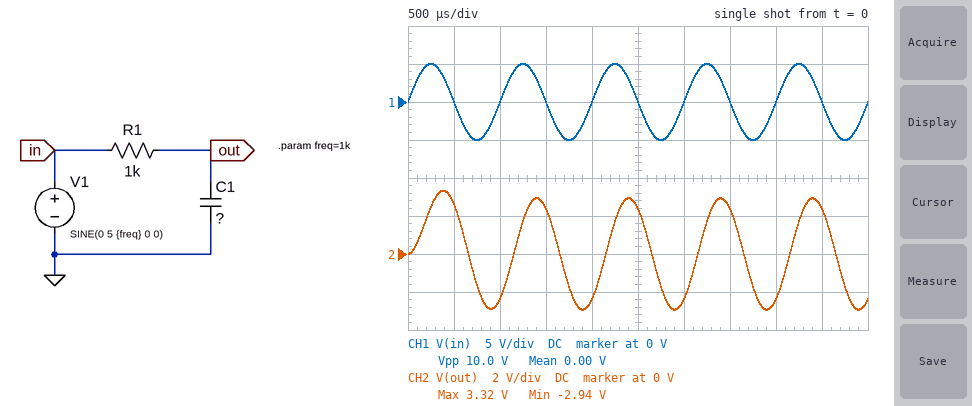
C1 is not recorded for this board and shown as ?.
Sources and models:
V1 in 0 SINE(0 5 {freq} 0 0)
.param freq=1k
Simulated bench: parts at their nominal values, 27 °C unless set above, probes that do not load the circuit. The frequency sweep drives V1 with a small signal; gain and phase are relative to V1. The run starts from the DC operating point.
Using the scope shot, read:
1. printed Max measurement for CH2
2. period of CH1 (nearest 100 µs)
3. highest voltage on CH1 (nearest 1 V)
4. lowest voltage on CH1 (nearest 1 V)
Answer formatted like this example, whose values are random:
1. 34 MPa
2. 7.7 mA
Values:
1. 3.32 V
2. 1.0 ms
3. 5 V
4. -5 V
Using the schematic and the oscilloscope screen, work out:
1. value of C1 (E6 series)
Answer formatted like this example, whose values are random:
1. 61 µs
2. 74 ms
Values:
1. 220 nF
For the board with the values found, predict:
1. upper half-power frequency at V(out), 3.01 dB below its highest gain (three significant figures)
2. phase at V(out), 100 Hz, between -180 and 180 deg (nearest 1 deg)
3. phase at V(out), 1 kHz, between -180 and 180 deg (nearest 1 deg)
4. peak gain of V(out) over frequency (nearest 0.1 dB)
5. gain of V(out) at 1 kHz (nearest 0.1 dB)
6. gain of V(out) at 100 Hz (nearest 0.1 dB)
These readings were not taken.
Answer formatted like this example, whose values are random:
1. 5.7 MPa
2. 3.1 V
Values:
1. 723 Hz
2. -8 deg
3. -54 deg
4. 0 dB
5. -4.6 dB
6. -0.1 dB
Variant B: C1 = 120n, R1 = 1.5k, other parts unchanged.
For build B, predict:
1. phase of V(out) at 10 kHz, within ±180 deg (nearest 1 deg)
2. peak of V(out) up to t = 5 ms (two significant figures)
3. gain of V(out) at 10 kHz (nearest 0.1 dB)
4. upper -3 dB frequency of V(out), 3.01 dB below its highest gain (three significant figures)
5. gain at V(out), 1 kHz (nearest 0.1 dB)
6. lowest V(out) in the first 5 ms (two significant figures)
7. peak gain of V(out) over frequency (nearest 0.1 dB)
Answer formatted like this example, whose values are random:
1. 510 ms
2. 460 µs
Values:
1. -85 deg
2. 3.6 V
3. -21.1 dB
4. 884 Hz
5. -3.6 dB
6. -3.3 V
7. 0 dB
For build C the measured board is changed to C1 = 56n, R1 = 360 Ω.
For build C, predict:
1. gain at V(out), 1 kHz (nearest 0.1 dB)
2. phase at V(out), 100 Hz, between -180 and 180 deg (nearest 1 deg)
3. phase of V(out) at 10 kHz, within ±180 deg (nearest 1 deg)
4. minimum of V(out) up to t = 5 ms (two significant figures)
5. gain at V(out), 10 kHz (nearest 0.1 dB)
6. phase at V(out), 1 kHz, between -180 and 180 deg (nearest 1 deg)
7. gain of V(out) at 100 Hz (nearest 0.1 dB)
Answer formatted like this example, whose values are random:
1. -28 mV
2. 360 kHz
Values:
1. -0.1 dB
2. -1 deg
3. -52 deg
4. -5.0 V
5. -4.2 dB
6. -7 deg
7. 0 dB
